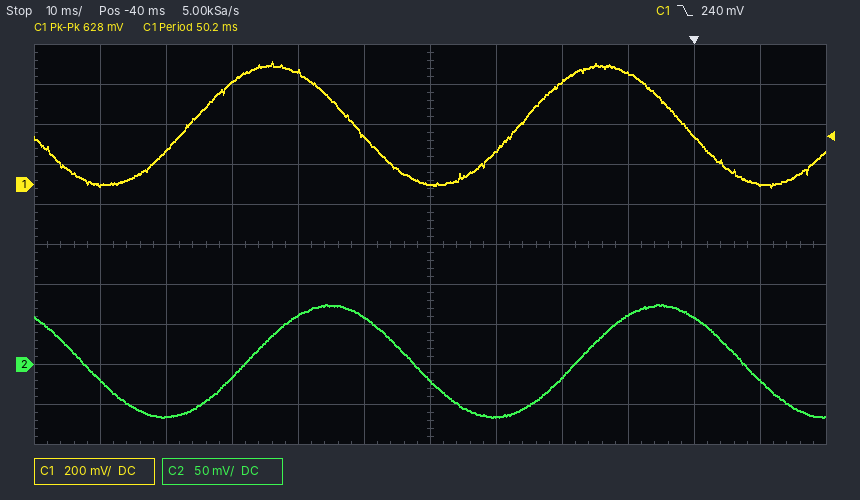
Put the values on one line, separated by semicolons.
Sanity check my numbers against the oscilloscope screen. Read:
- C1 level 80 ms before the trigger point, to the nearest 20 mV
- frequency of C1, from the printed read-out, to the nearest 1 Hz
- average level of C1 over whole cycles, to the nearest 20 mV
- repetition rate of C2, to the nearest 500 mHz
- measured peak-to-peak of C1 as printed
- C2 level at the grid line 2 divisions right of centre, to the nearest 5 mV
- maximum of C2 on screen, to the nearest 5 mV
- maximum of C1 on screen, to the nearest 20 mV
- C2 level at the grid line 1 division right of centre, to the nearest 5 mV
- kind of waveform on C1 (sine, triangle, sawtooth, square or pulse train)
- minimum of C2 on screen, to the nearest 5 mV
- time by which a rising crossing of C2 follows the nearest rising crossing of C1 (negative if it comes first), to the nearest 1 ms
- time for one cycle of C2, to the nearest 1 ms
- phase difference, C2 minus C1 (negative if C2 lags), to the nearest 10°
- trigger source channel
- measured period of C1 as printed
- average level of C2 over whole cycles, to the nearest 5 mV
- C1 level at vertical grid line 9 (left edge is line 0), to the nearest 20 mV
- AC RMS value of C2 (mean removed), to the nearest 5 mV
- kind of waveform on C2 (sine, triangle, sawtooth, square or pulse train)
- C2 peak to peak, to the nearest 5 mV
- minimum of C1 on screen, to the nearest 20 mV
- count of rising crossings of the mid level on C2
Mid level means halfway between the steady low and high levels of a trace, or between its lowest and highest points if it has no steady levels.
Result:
160 mV; 20 Hz; 300 mV; 20.0 Hz; 628 mV; -15 mV; 75 mV; 620 mV; -65 mV; sine; -65 mV; +9 ms; 50 ms; -60°; C1; 50.2 ms; 5 mV; 560 mV; 50 mV; sine; 140 mV; -20 mV; 2
